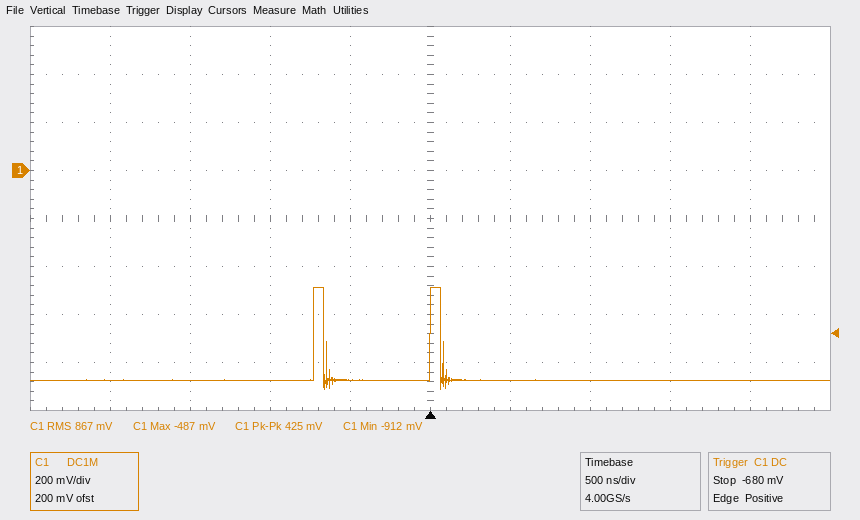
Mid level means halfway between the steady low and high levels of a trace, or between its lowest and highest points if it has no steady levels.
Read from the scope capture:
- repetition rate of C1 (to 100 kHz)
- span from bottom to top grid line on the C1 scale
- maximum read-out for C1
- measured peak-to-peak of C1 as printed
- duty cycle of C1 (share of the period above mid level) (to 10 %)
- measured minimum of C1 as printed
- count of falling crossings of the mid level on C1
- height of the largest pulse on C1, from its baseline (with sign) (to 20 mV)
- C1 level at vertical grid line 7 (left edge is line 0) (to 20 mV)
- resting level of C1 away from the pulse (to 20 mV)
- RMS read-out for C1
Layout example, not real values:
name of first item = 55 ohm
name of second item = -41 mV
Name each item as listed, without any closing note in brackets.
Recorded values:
repetition rate of C1 = 1.4 MHz
span from bottom to top grid line on the C1 scale = 1.6 V
maximum read-out for C1 = -487 mV
measured peak-to-peak of C1 as printed = 425 mV
duty cycle of C1 (share of the period above mid level) = 10 %
measured minimum of C1 as printed = -912 mV
count of falling crossings of the mid level on C1 = 2
height of the largest pulse on C1, from its baseline (with sign) = +380 mV
C1 level at vertical grid line 7 (left edge is line 0) = -880 mV
resting level of C1 away from the pulse = -880 mV
RMS read-out for C1 = 867 mV
